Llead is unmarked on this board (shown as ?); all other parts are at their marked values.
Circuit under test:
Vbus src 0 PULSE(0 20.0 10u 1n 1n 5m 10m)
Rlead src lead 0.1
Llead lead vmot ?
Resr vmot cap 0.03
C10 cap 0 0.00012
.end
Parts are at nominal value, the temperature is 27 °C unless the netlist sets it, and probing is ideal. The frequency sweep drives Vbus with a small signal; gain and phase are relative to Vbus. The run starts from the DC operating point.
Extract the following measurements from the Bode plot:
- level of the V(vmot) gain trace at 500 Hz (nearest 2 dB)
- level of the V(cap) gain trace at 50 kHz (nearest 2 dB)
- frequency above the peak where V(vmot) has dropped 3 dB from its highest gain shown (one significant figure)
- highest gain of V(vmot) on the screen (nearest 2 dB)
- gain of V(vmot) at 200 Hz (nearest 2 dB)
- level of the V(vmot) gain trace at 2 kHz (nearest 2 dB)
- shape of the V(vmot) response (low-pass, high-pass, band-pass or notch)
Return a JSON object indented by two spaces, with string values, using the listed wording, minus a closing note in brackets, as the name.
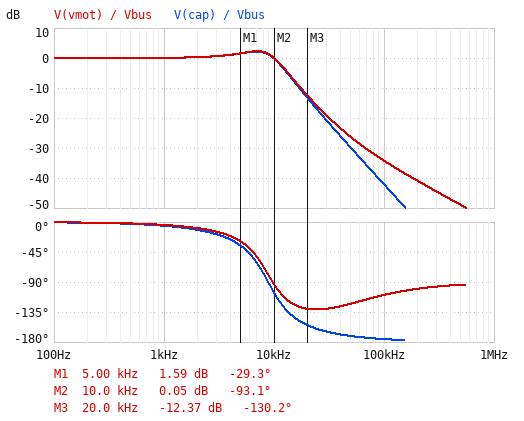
{
  "level of the V(vmot) gain trace at 500 Hz": "0 dB",
  "level of the V(cap) gain trace at 50 kHz": "-30 dB",
  "frequency above the peak where V(vmot) has dropped 3 dB from its highest gain shown": "10 kHz",
  "highest gain of V(vmot) on the screen": "2 dB",
  "gain of V(vmot) at 200 Hz": "0 dB",
  "level of the V(vmot) gain trace at 2 kHz": "0 dB",
  "shape of the V(vmot) response": "low-pass"
}
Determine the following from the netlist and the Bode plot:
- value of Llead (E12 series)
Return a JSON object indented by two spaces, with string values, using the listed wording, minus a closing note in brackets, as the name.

{
  "value of Llead": "2.7 µH"
}
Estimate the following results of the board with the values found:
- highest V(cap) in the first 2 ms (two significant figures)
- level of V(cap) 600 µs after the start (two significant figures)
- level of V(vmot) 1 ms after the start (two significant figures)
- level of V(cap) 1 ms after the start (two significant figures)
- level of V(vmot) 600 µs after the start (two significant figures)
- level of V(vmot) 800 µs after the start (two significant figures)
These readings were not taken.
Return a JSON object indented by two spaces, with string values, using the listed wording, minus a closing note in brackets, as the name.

{
  "highest V(cap) in the first 2 ms": "24 V",
  "level of V(cap) 600 µs after the start": "20 V",
  "level of V(vmot) 1 ms after the start": "20 V",
  "level of V(cap) 1 ms after the start": "20 V",
  "level of V(vmot) 600 µs after the start": "20 V",
  "level of V(vmot) 800 µs after the start": "20 V"
}
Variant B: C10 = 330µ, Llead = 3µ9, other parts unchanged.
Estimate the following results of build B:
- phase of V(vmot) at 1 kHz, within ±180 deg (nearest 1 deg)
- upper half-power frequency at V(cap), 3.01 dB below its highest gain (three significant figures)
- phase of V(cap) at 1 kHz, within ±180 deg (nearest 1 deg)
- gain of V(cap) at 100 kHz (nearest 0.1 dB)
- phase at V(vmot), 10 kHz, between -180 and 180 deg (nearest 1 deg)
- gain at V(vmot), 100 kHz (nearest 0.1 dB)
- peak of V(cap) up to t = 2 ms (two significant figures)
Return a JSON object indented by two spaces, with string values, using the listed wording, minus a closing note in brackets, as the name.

{
  "phase of V(vmot) at 1 kHz, within ±180 deg": "-12 deg",
  "upper half-power frequency at V(cap), 3.01 dB below its highest gain": "4.95 kHz",
  "phase of V(cap) at 1 kHz, within ±180 deg": "-16 deg",
  "gain of V(cap) at 100 kHz": "-54.1 dB",
  "phase at V(vmot), 10 kHz, between -180 and 180 deg": "-115 deg",
  "gain at V(vmot), 100 kHz": "-38.1 dB",
  "peak of V(cap) up to t = 2 ms": "22 V"
}
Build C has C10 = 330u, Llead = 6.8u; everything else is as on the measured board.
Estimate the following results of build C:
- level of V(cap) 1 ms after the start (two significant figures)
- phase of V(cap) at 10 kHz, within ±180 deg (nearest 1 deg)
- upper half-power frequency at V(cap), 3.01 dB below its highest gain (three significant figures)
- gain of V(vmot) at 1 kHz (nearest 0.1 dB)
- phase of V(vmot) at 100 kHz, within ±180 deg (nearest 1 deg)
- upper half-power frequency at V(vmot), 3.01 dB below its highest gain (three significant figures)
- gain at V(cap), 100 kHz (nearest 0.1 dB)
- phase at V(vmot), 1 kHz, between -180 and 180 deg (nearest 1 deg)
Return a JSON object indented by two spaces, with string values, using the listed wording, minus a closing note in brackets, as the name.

{
  "level of V(cap) 1 ms after the start": "20 V",
  "phase of V(cap) at 10 kHz, within ±180 deg": "-161 deg",
  "upper half-power frequency at V(cap), 3.01 dB below its highest gain": "3.97 kHz",
  "gain of V(vmot) at 1 kHz": "0.5 dB",
  "phase of V(vmot) at 100 kHz, within ±180 deg": "-97 deg",
  "upper half-power frequency at V(vmot), 3.01 dB below its highest gain": "4.01 kHz",
  "gain at V(cap), 100 kHz": "-58.9 dB",
  "phase at V(vmot), 1 kHz, between -180 and 180 deg": "-13 deg"
}
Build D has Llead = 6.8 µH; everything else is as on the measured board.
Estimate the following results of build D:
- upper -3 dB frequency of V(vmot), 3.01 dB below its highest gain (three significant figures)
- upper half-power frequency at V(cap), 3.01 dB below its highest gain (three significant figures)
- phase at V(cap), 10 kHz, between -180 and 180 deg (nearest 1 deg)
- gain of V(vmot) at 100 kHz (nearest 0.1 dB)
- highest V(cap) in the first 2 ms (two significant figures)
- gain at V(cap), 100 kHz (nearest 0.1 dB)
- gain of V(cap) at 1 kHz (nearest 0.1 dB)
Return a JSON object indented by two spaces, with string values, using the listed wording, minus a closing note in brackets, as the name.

{
  "upper -3 dB frequency of V(vmot), 3.01 dB below its highest gain": "6.55 kHz",
  "upper half-power frequency at V(cap), 3.01 dB below its highest gain": "6.54 kHz",
  "phase at V(cap), 10 kHz, between -180 and 180 deg": "-156 deg",
  "gain of V(vmot) at 100 kHz": "-42.3 dB",
  "highest V(cap) in the first 2 ms": "28 V",
  "gain at V(cap), 100 kHz": "-50.1 dB",
  "gain of V(cap) at 1 kHz": "0.2 dB"
}
